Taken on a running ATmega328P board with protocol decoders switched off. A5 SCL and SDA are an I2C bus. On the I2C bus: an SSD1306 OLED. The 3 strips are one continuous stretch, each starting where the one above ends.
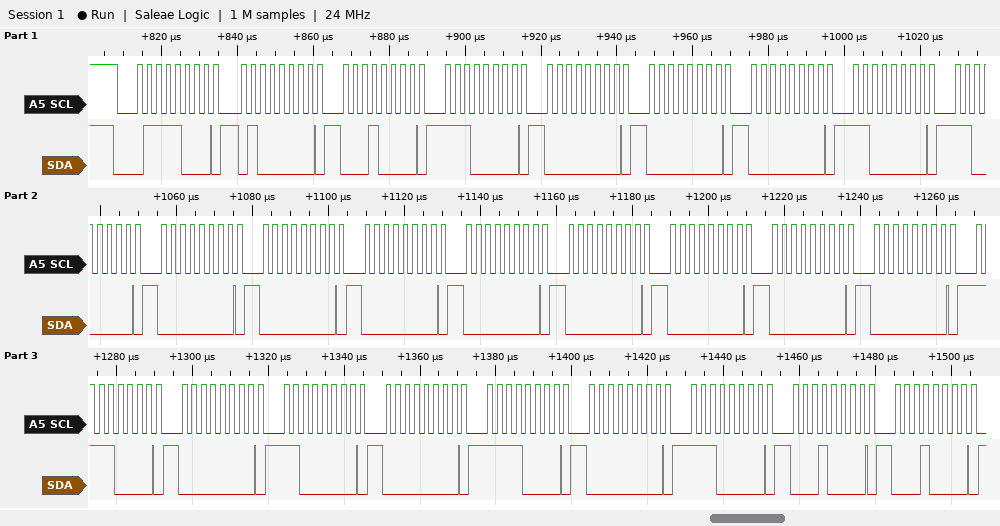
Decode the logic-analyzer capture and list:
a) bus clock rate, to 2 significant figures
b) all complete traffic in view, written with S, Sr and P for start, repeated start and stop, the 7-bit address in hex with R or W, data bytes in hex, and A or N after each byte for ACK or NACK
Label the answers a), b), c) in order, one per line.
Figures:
a) 400 kHz
b) S 3CW A 40 A 10 A E0 A 00 A 00 A 00 A C0 A C0 A 00 A 00 A 00 A 00 A 00 A 00 A 00 A 00 A F0 A 00 A C0 A 00 A F0 A 00 A E0 A 10 A 10 A
